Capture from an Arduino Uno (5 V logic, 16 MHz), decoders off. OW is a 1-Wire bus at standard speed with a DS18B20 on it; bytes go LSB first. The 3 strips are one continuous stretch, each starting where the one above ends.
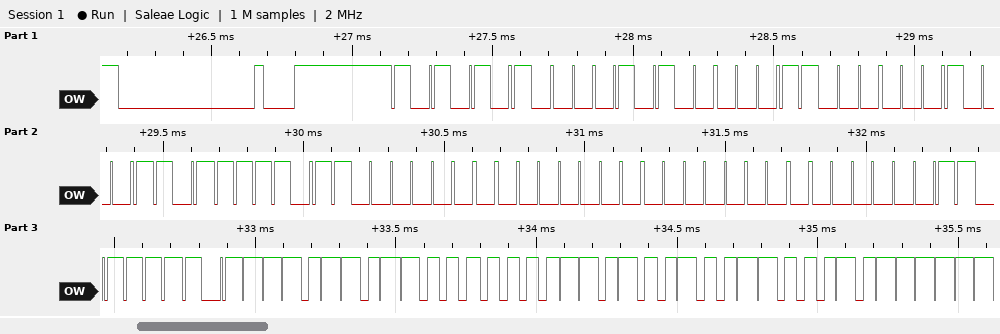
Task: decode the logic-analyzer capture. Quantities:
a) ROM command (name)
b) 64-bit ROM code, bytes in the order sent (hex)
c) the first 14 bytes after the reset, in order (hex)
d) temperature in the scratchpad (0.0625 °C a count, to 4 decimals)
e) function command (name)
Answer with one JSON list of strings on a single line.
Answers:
["Match ROM", "28 18 88 7D 03 00 00 C0", "55 28 18 88 7D 03 00 00 C0 BE B7 01 4B 46", "27.4375 °C", "Read Scratchpad"]
